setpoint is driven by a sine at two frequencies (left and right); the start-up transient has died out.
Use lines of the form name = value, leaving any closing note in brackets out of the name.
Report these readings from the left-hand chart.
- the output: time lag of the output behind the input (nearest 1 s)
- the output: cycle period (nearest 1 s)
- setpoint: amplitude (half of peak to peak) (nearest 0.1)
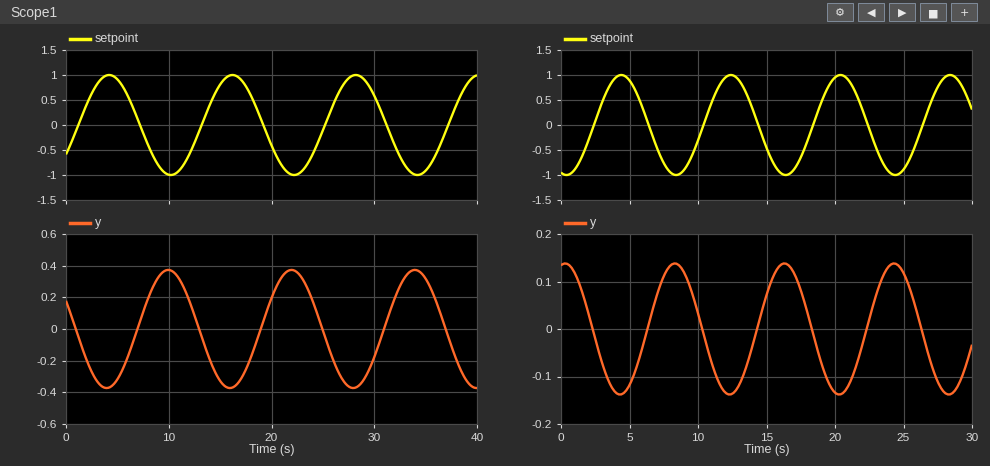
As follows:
the output: time lag of the output behind the input = 6 s
the output: cycle period = 12 s
setpoint: amplitude (half of peak to peak) = 1.0
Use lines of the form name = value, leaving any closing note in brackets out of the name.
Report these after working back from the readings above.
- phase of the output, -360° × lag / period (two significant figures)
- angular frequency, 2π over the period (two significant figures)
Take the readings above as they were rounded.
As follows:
phase of the output, -360° × lag / period = -180°
angular frequency, 2π over the period = 0.52 rad/s
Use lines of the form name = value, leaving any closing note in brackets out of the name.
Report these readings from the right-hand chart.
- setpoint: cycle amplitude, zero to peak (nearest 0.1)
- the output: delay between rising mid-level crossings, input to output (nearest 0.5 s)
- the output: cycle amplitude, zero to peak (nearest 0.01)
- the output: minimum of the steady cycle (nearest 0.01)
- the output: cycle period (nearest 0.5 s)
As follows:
setpoint: cycle amplitude, zero to peak = 1.0
the output: delay between rising mid-level crossings, input to output = 4.0 s
the output: cycle amplitude, zero to peak = 0.14
the output: minimum of the steady cycle = -0.14
the output: cycle period = 8.0 s
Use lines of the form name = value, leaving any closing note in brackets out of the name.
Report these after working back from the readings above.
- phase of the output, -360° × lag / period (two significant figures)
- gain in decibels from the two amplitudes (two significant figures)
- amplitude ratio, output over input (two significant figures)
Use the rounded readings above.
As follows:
phase of the output, -360° × lag / period = -180°
gain in decibels from the two amplitudes = -17 dB
amplitude ratio, output over input = 0.14
